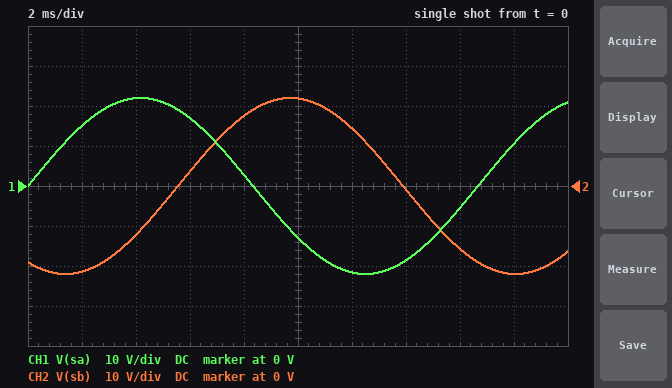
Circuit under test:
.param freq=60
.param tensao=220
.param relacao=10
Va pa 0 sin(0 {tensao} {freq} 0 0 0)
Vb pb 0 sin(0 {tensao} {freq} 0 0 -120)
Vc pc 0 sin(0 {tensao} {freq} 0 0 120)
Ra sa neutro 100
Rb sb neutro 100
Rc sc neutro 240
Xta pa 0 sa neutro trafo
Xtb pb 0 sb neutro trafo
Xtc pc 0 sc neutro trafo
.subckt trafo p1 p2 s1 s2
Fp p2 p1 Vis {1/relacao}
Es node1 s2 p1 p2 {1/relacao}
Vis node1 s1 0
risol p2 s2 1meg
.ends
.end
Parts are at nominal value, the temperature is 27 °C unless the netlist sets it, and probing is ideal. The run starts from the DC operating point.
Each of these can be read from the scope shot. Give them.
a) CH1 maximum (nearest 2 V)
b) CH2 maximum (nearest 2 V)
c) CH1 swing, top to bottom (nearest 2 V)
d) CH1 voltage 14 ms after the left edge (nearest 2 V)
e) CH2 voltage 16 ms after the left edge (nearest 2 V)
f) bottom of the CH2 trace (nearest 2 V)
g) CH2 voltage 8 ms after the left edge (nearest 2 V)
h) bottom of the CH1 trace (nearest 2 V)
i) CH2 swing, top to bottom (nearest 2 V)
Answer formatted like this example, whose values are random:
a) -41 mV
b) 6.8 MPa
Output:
a) 22 V
b) 22 V
c) 44 V
d) -18 V
e) -16 V
f) -22 V
g) 18 V
h) -22 V
i) 44 V
